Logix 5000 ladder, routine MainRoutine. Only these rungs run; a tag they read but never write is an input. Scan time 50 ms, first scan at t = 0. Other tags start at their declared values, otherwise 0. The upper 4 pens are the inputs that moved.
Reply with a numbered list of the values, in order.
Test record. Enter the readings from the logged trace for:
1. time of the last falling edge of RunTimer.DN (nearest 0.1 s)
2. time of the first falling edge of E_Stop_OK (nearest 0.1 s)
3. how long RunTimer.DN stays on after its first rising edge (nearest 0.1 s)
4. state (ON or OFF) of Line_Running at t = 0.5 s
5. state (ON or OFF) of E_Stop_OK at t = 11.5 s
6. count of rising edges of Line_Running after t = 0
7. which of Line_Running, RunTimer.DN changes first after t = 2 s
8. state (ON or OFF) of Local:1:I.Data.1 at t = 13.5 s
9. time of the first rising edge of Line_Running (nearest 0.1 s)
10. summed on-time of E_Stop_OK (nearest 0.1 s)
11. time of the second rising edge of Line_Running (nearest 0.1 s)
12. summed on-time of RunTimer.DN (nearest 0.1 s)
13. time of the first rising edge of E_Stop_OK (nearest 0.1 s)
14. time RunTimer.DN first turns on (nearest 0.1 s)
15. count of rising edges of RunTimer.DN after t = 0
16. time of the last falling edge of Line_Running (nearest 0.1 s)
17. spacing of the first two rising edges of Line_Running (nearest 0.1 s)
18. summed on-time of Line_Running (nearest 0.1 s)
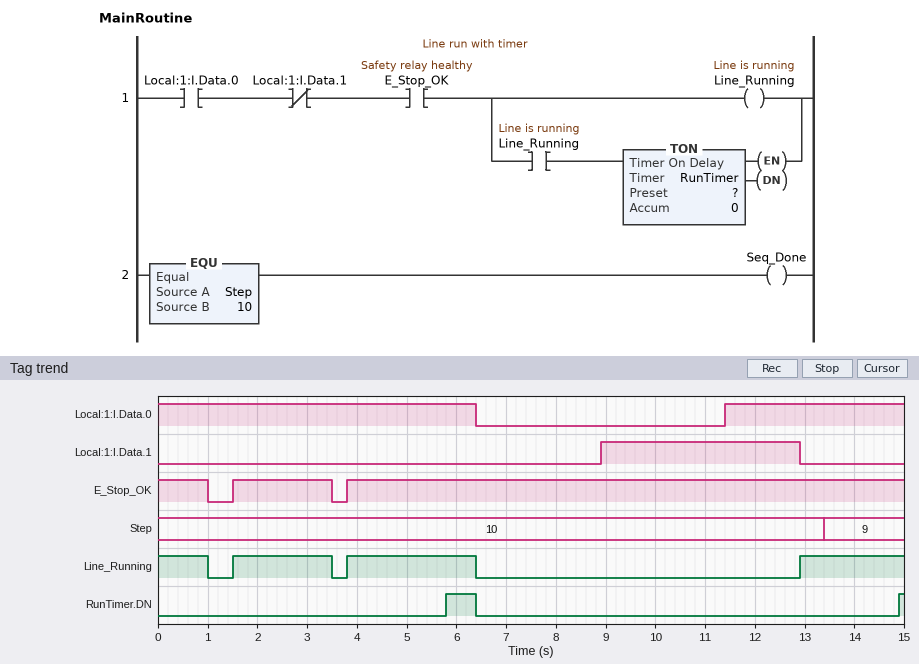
1. 6.4 s
2. 1.0 s
3. 0.6 s
4. ON
5. ON
6. 3
7. Line_Running
8. OFF
9. 1.5 s
10. 14.2 s
11. 3.8 s
12. 0.7 s
13. 1.5 s
14. 5.8 s
15. 2
16. 6.4 s
17. 2.3 s
18. 7.7 s
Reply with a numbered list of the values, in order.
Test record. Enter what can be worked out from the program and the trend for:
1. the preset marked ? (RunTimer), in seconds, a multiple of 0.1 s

1. 2.0 s
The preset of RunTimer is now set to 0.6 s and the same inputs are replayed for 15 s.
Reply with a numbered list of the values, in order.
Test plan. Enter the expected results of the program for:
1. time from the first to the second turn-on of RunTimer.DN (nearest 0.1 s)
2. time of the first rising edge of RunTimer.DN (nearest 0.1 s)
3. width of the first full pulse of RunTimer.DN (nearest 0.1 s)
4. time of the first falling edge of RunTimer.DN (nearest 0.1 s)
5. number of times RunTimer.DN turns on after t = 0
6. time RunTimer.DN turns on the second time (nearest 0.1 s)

1. 1.5 s
2. 0.6 s
3. 0.4 s
4. 1.0 s
5. 4
6. 2.1 s
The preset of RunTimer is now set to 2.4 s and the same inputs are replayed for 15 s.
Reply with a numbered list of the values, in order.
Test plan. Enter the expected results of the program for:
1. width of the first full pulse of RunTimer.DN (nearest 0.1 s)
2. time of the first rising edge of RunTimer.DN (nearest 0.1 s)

1. 0.2 s
2. 6.2 s
